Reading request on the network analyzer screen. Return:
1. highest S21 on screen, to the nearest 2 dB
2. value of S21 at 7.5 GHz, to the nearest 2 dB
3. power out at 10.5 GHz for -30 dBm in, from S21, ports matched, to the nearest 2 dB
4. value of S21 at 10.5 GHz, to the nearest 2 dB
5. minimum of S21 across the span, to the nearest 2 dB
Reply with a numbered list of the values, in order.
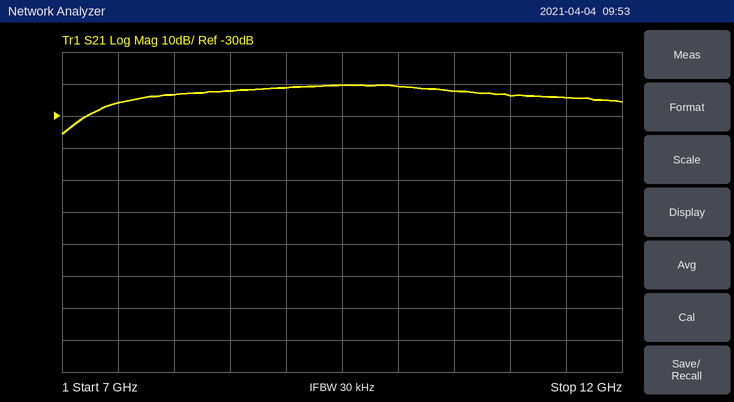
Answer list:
1. -20 dB
2. -26 dB
3. -52 dBm
4. -22 dB
5. -36 dB
